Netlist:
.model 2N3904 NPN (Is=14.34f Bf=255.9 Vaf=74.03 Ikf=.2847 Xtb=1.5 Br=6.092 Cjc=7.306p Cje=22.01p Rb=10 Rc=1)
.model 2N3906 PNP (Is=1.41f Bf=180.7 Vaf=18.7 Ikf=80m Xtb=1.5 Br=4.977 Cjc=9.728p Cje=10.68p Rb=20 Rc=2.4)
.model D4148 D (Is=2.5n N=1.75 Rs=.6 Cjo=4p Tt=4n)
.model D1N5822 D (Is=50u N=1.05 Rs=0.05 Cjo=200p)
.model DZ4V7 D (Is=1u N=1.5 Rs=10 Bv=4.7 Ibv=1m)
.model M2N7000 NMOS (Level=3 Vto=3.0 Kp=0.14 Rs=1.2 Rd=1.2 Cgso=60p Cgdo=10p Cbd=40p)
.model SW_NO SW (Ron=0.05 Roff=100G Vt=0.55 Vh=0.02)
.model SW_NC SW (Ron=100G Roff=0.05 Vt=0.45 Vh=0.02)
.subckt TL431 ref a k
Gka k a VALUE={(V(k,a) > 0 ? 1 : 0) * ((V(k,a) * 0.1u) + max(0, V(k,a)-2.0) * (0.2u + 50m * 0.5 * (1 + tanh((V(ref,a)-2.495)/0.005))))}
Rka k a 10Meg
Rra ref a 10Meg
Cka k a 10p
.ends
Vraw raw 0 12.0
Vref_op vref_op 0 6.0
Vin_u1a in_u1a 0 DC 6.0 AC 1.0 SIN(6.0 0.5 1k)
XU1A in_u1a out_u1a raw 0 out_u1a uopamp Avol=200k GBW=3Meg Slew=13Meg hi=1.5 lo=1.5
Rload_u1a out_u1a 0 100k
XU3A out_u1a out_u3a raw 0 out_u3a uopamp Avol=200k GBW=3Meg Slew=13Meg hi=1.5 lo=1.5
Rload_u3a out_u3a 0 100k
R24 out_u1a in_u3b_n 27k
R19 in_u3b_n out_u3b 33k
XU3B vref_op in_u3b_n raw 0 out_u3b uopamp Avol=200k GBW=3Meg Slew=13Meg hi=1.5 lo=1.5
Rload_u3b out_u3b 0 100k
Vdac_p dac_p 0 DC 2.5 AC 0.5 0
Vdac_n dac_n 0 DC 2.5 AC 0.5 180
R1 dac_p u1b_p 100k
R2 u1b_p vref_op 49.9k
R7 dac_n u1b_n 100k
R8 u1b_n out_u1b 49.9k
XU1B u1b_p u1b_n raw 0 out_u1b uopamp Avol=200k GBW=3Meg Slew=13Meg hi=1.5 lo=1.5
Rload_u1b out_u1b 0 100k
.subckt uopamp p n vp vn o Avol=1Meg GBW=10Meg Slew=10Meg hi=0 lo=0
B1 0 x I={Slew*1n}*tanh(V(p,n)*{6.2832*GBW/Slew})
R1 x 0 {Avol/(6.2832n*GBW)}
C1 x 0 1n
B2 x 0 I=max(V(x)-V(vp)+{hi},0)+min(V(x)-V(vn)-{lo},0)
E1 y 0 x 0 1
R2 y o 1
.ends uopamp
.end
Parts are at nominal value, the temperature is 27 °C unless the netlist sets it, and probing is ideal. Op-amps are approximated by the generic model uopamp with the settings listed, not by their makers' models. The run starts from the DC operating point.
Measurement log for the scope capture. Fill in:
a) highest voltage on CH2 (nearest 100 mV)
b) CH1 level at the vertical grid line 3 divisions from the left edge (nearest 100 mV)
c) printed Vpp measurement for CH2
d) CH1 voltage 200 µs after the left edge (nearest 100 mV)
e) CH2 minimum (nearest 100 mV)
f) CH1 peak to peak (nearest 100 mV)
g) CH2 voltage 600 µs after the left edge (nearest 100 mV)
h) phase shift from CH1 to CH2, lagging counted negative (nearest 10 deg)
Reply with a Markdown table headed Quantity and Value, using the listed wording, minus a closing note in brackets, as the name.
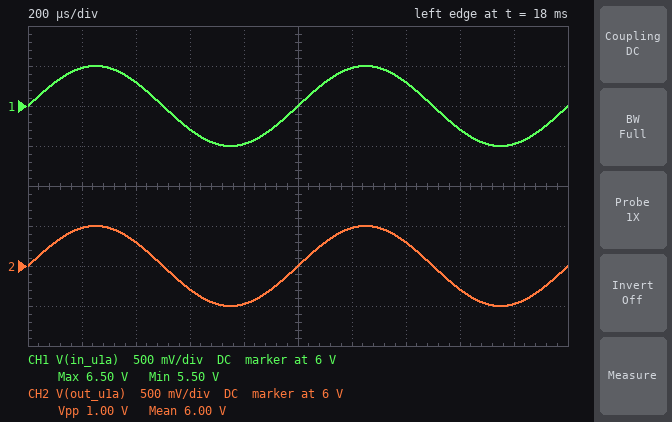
| Quantity | Value |
|---|---|
| highest voltage on CH2 | 6.5 V |
| CH1 level at the vertical grid line 3 divisions from the left edge | 5.7 V |
| printed Vpp measurement for CH2 | 1.00 V |
| CH1 voltage 200 µs after the left edge | 6.5 V |
| CH2 minimum | 5.5 V |
| CH1 peak to peak | 1.0 V |
| CH2 voltage 600 µs after the left edge | 5.7 V |
| phase shift from CH1 to CH2, lagging counted negative | 0 deg |
